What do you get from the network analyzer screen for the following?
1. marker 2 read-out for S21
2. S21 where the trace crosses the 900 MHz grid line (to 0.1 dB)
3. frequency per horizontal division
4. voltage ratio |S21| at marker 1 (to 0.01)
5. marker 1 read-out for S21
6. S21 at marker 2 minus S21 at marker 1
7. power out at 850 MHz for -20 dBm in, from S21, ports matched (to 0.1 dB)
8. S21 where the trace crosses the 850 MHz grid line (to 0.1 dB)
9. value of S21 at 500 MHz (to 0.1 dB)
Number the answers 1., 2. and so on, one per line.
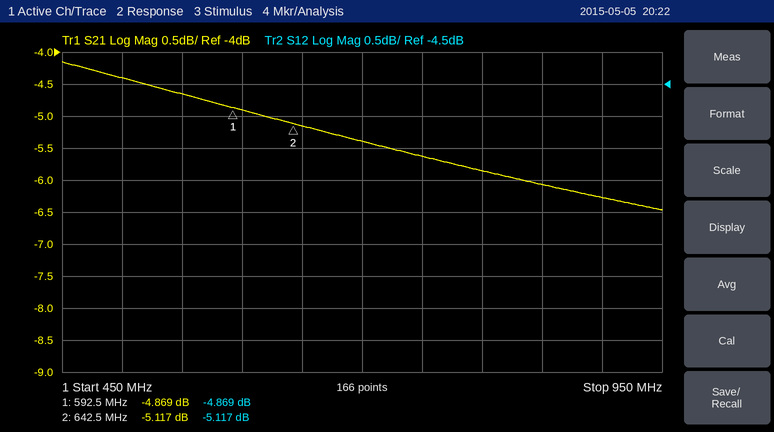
1. -5.117 dB
2. -6.3 dB
3. 50 MHz
4. 0.57
5. -4.869 dB
6. -0.248 dB
7. -26.1 dBm
8. -6.1 dB
9. -4.4 dB
